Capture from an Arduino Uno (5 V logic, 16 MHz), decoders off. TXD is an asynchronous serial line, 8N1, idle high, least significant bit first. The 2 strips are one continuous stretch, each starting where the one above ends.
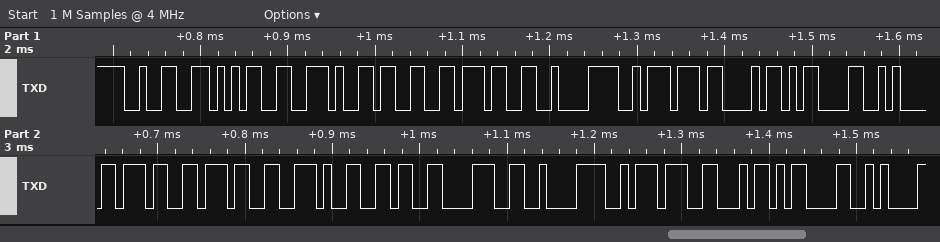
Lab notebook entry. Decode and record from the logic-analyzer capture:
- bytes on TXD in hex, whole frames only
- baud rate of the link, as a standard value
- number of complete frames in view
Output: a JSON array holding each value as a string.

["32 35 2E 33 37 C2 BA 43 0D 0A 37 37 2E 36 38 C2 BA 46 0D 0A", "115200 baud", "20"]
